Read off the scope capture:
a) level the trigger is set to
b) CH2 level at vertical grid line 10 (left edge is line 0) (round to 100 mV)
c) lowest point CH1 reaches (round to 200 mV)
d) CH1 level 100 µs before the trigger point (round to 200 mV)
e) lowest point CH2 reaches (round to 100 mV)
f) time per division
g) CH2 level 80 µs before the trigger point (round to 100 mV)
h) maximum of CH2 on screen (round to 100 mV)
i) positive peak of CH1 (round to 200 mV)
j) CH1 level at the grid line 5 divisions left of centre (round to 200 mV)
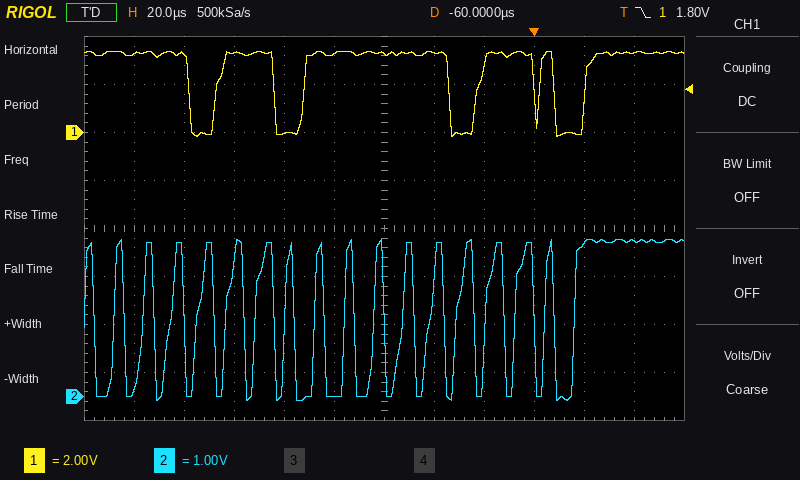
1.80 V
3.2 V
-200 mV
0.0 V
-100 mV
20 µs
0.0 V
3.3 V
3.4 V
3.2 V
